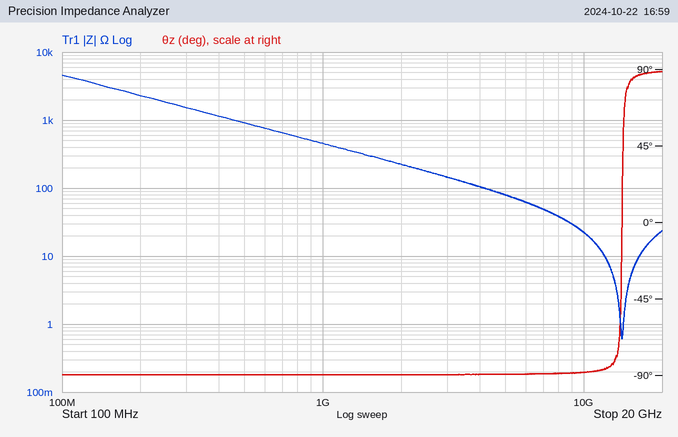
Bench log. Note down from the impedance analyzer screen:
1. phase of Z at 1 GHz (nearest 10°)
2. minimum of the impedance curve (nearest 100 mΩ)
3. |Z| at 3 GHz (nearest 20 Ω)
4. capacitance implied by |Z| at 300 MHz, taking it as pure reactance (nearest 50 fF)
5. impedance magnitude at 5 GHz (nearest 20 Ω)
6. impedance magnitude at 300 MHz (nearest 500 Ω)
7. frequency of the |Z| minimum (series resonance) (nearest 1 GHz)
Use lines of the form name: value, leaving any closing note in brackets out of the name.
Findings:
phase of Z at 1 GHz: -90°
minimum of the impedance curve: 600 mΩ
|Z| at 3 GHz: 140 Ω
capacitance implied by |Z| at 300 MHz, taking it as pure reactance: 350 fF
impedance magnitude at 5 GHz: 80 Ω
impedance magnitude at 300 MHz: 1.5 kΩ
frequency of the |Z| minimum (series resonance): 14 GHz
